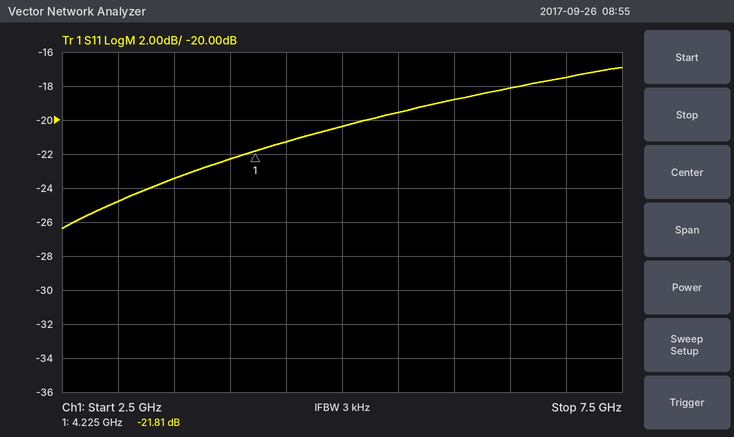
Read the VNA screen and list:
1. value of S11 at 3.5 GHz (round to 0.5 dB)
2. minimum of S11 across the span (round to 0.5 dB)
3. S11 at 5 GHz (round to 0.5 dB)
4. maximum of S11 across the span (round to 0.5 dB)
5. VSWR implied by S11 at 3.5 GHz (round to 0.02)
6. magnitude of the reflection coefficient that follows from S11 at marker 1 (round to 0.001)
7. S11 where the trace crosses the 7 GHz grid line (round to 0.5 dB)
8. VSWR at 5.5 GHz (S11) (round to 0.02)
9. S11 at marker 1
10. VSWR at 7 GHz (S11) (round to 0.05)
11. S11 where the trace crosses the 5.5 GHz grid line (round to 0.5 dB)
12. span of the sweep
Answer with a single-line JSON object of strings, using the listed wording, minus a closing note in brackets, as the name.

{"value of S11 at 3.5 GHz": "-23.5 dB", "minimum of S11 across the span": "-26.5 dB", "S11 at 5 GHz": "-20.5 dB", "maximum of S11 across the span": "-17.0 dB", "VSWR implied by S11 at 3.5 GHz": "1.14", "magnitude of the reflection coefficient that follows from S11 at marker 1": "0.081", "S11 where the trace crosses the 7 GHz grid line": "-17.5 dB", "VSWR at 5.5 GHz (S11)": "1.24", "S11 at marker 1": "-21.81 dB", "VSWR at 7 GHz (S11)": "1.30", "S11 where the trace crosses the 5.5 GHz grid line": "-19.5 dB", "span of the sweep": "5 GHz"}
